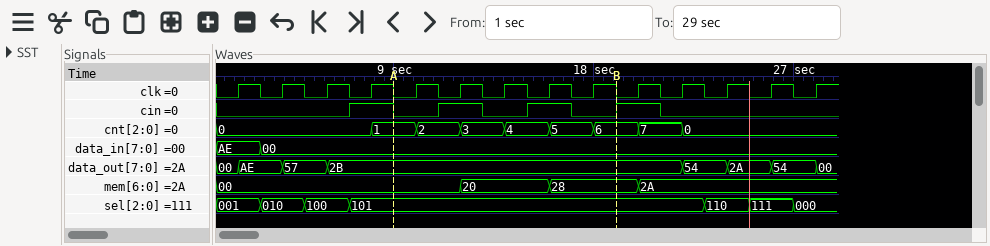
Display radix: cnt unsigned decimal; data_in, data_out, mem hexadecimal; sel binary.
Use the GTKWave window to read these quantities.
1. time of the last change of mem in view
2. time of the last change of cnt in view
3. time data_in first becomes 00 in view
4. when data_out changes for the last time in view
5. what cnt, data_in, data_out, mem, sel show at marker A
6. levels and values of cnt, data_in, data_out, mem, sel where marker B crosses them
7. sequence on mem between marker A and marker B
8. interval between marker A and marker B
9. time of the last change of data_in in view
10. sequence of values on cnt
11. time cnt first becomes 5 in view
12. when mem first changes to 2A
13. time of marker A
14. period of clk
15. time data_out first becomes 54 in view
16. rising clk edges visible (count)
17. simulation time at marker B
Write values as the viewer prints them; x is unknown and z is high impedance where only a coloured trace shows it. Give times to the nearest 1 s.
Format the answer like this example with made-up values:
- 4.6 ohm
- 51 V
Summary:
- 20 s
- 22 s
- 3 s
- 28 s
- cnt=1, data_in=00, data_out=2B, mem=00, sel=101
- cnt=6, data_in=00, data_out=2B, mem=28, sel=101
- 00, 20, 28
- 10 s
- 3 s
- 0, 1, 2, 3, 4, 5, 6, 7, 0
- 16 s
- 20 s
- 9 s
- 2 s
- 22 s
- 14
- 19 s
